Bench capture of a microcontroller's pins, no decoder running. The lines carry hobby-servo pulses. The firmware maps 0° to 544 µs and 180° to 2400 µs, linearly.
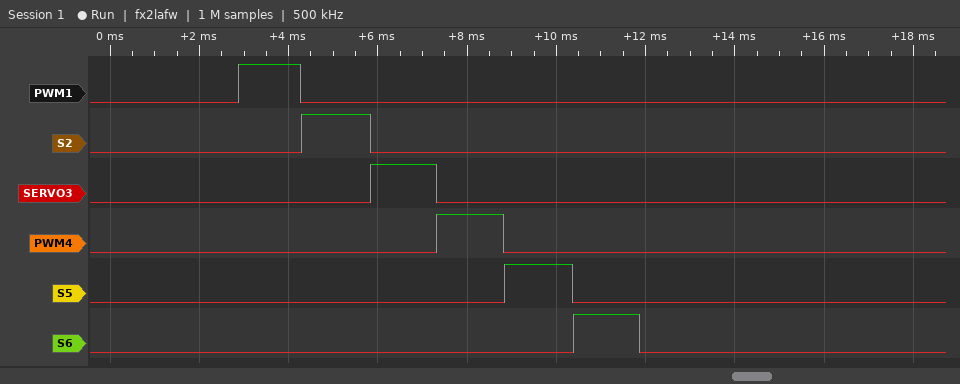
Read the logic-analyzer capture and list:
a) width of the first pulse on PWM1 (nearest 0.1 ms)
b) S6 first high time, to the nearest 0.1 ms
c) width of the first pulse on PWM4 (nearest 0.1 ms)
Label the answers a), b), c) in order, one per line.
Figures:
a) 1.4 ms
b) 1.5 ms
c) 1.5 ms
